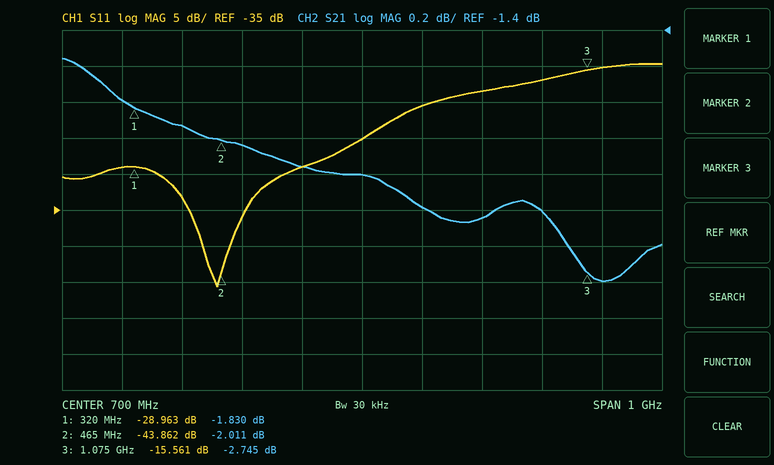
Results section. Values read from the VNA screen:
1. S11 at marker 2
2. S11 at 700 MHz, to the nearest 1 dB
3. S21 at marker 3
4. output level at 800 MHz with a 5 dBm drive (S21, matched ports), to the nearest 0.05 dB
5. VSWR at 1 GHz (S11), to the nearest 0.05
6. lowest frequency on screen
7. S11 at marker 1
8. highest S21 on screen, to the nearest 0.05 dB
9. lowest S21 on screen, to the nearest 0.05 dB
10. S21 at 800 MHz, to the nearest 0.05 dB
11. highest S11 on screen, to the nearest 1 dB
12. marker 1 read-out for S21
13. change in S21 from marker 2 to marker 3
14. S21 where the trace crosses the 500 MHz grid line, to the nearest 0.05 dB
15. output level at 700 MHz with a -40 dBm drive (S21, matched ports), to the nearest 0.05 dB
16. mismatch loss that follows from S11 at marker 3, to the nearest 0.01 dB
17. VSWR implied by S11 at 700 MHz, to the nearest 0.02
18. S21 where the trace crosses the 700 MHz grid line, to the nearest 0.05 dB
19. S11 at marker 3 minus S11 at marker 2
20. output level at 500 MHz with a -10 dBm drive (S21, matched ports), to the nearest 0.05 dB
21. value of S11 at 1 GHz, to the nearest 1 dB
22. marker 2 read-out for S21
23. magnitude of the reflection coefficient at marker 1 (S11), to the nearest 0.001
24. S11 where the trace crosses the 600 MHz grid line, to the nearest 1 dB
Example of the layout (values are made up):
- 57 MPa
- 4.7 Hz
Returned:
- -43.862 dB
- -25 dB
- -2.745 dB
- 2.60 dBm
- 1.35
- 200 MHz
- -28.963 dB
- -1.55 dB
- -2.80 dB
- -2.40 dB
- -15 dB
- -1.830 dB
- -0.734 dB
- -2.05 dB
- -42.20 dBm
- 0.12 dB
- 1.12
- -2.20 dB
- 28.301 dB
- -12.05 dBm
- -17 dB
- -2.011 dB
- 0.036
- -29 dB
